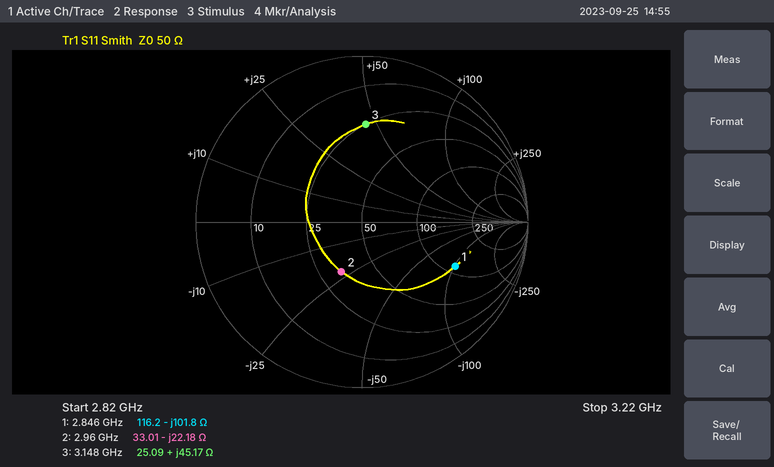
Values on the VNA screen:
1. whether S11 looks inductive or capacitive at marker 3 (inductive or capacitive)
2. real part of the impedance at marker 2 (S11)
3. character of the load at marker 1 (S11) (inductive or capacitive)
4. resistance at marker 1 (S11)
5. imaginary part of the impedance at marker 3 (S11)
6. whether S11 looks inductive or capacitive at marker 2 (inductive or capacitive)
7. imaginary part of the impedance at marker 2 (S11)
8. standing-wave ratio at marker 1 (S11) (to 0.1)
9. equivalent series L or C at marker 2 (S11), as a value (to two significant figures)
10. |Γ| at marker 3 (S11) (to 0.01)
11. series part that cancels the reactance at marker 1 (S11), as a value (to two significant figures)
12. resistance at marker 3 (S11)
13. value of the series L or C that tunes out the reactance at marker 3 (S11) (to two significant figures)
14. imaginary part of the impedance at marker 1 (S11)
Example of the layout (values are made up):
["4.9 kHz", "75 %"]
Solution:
["inductive", "33.01 Ω", "capacitive", "116.2 Ω", "+45.17 Ω", "capacitive", "-22.18 Ω", "4.3", "2.4 pF", "0.59", "5.7 nH", "25.09 Ω", "1.1 pF", "-101.8 Ω"]
